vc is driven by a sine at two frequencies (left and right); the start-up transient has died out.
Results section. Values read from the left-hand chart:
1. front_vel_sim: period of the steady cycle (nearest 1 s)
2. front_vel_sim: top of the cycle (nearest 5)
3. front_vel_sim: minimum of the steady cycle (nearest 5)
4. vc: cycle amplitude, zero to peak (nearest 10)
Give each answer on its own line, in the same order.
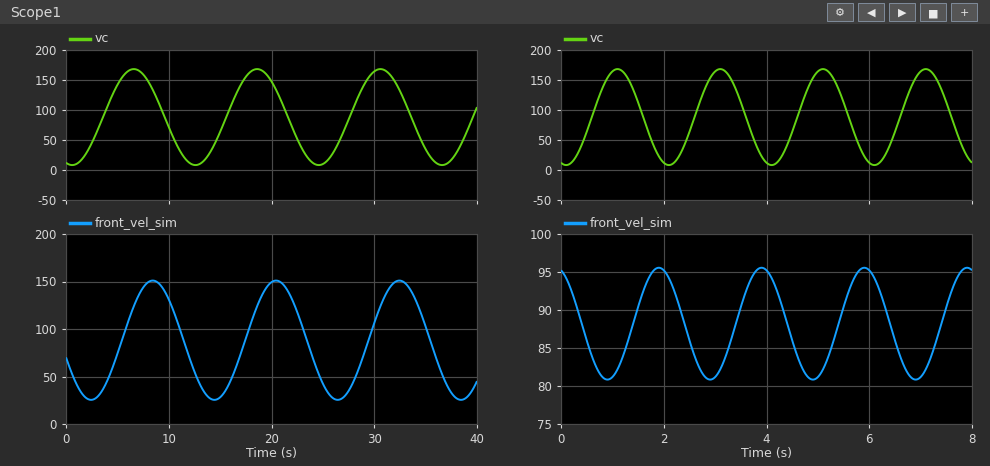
12 s
150
25
80
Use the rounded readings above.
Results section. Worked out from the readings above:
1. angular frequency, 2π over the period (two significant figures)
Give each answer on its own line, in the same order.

0.52 rad/s
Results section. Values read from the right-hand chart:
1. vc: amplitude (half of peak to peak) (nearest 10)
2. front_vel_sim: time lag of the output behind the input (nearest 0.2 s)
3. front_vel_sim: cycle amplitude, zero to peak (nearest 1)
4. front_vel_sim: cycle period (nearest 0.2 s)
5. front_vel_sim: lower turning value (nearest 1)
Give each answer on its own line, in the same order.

80
0.8 s
7
2.0 s
81
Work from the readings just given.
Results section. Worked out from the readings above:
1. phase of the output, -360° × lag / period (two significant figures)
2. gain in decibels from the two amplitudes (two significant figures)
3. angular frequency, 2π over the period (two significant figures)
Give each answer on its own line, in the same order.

-140°
-21 dB
3.1 rad/s
